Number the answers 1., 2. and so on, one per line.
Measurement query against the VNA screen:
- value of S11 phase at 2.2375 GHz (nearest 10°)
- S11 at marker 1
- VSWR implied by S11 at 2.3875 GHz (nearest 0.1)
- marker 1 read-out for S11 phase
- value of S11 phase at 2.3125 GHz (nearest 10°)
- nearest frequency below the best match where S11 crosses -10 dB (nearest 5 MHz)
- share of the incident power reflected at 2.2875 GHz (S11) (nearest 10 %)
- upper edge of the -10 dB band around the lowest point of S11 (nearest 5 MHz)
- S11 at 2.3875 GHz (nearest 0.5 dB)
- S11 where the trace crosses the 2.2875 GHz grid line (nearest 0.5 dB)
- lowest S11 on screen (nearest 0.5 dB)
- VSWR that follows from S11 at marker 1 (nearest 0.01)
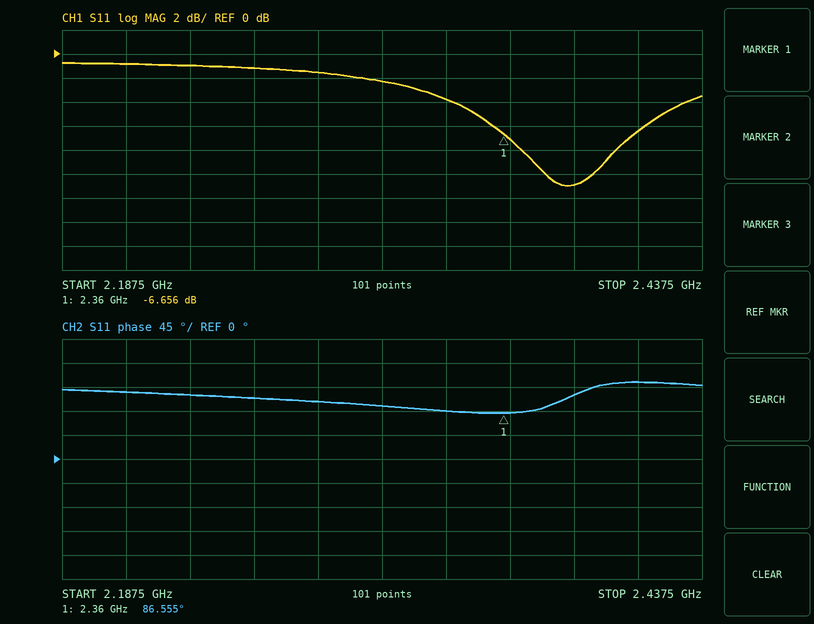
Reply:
1. 120°
2. -6.656 dB
3. 1.8
4. 86.555°
5. 100°
6. 2.375 GHz
7. 70 %
8. 2.395 GHz
9. -11.0 dB
10. -1.5 dB
11. -11.0 dB
12. 2.74
